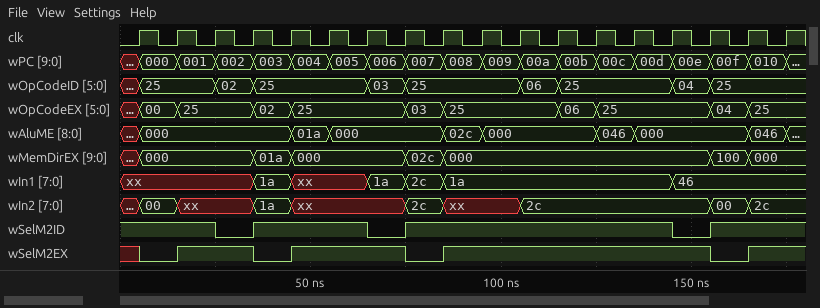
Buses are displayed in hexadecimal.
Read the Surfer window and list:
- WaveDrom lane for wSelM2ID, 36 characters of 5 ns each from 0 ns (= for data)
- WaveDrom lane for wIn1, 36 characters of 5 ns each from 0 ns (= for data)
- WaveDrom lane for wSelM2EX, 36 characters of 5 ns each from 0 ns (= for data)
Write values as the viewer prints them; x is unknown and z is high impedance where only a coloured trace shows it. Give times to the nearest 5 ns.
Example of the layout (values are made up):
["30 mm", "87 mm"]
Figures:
["{name: 'wSelM2ID', wave: '1....0.1.....0.1.............0.1....'}", "{name: 'wIn1', wave: 'x......=.x...=.=.=...........=......', data: '1a 1a 2c 1a 46'}", "{name: 'wSelM2EX', wave: 'x0.1...0.1.....0.1.............0.1..'}"]
